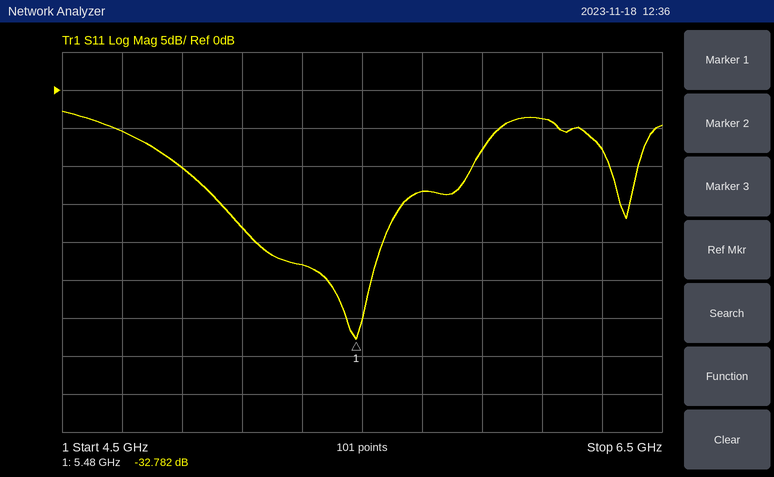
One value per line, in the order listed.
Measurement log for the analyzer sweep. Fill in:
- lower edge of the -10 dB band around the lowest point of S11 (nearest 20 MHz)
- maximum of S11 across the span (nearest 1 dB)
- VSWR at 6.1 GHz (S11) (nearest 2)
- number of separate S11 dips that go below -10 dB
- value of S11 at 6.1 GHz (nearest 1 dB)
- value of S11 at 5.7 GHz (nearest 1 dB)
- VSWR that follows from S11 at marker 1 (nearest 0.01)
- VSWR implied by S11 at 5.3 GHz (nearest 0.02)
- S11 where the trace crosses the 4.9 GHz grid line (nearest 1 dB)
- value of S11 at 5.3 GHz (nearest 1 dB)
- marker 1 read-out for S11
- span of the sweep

4.90 GHz
-3 dB
4
2
-4 dB
-13 dB
1.05
1.16
-10 dB
-23 dB
-32.782 dB
2 GHz
